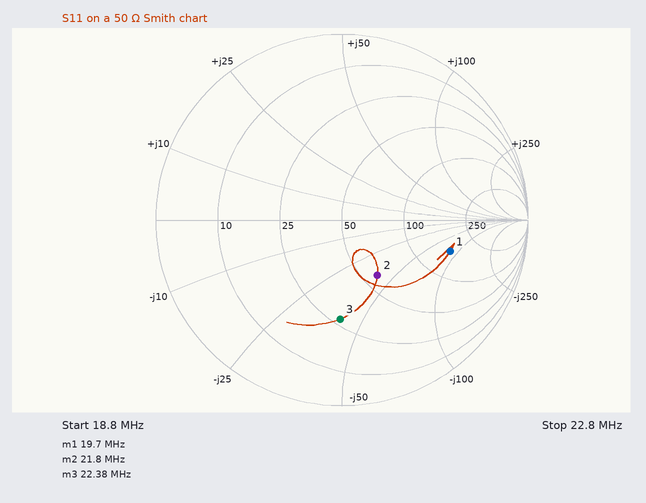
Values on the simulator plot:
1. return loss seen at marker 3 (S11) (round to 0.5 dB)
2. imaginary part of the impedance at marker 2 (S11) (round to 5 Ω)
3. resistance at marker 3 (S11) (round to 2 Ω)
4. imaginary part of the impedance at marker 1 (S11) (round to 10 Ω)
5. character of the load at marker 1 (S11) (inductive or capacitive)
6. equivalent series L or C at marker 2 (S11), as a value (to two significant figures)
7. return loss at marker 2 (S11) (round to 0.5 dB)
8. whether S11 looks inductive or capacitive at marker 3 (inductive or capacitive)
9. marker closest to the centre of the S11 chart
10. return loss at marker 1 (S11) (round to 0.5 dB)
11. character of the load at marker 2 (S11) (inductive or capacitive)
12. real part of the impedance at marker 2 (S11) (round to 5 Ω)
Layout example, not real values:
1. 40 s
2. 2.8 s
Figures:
1. 5.5 dB
2. -40 Ω
3. 28 Ω
4. -80 Ω
5. capacitive
6. 180 pF
7. 9.0 dB
8. capacitive
9. marker 2
10. 4.5 dB
11. capacitive
12. 60 Ω
